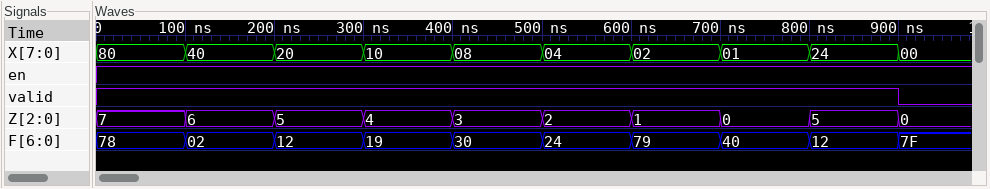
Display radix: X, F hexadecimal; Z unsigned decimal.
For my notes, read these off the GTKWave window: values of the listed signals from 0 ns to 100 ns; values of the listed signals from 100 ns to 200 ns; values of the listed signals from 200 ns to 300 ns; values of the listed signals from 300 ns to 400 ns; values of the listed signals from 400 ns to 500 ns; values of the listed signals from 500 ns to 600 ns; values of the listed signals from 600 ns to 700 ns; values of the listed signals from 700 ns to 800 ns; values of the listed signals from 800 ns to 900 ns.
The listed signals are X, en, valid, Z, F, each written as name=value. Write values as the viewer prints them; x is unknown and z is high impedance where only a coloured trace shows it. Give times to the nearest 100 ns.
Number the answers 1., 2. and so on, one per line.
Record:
1. X=80, en=1, valid=1, Z=7, F=78
2. X=40, en=1, valid=1, Z=6, F=02
3. X=20, en=1, valid=1, Z=5, F=12
4. X=10, en=1, valid=1, Z=4, F=19
5. X=08, en=1, valid=1, Z=3, F=30
6. X=04, en=1, valid=1, Z=2, F=24
7. X=02, en=1, valid=1, Z=1, F=79
8. X=01, en=1, valid=1, Z=0, F=40
9. X=24, en=1, valid=1, Z=5, F=12
